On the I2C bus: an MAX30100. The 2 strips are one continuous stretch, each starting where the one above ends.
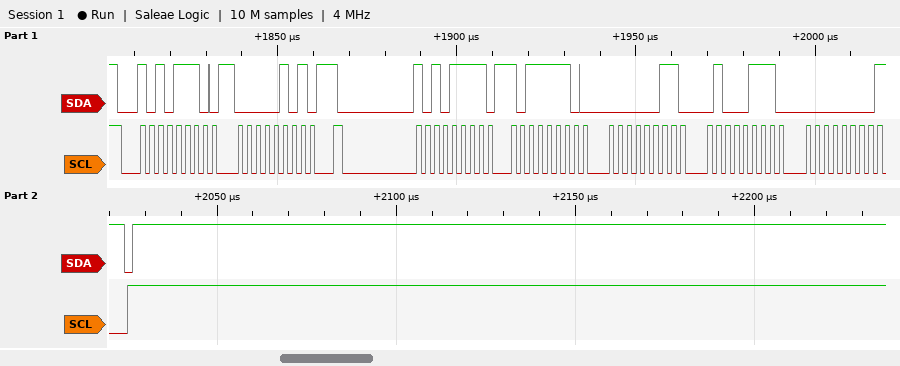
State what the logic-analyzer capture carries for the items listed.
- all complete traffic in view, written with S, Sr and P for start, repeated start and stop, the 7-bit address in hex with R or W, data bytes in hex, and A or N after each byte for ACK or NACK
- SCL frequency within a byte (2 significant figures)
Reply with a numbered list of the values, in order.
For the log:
1. S 57W A 05 A Sr 57R A BE A 03 A 47 A 00 N P
2. 400 kHz
